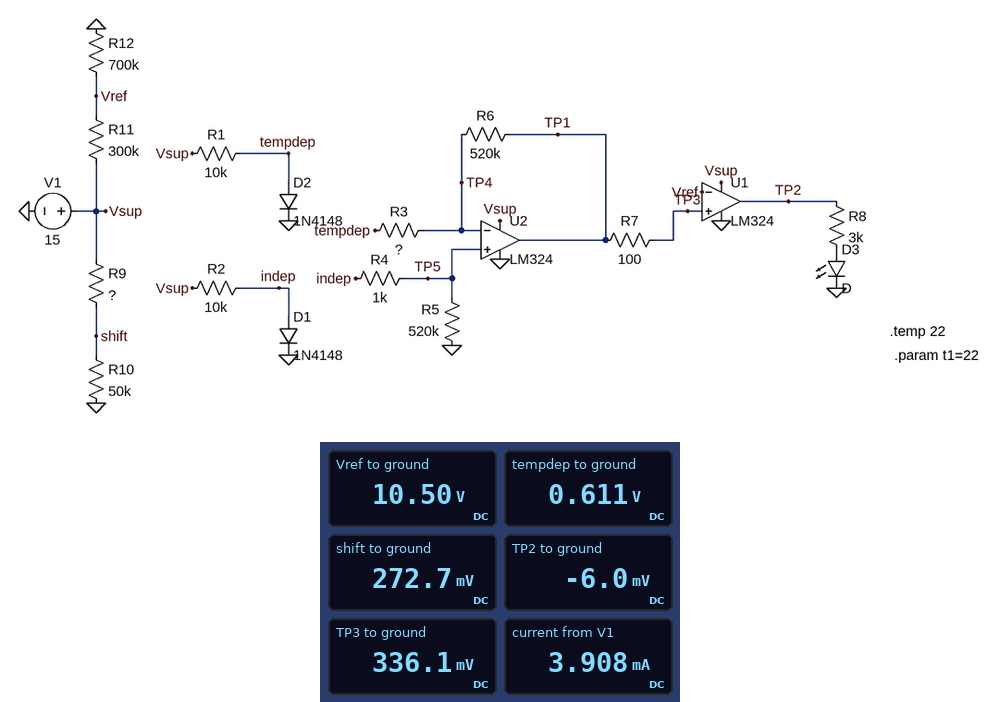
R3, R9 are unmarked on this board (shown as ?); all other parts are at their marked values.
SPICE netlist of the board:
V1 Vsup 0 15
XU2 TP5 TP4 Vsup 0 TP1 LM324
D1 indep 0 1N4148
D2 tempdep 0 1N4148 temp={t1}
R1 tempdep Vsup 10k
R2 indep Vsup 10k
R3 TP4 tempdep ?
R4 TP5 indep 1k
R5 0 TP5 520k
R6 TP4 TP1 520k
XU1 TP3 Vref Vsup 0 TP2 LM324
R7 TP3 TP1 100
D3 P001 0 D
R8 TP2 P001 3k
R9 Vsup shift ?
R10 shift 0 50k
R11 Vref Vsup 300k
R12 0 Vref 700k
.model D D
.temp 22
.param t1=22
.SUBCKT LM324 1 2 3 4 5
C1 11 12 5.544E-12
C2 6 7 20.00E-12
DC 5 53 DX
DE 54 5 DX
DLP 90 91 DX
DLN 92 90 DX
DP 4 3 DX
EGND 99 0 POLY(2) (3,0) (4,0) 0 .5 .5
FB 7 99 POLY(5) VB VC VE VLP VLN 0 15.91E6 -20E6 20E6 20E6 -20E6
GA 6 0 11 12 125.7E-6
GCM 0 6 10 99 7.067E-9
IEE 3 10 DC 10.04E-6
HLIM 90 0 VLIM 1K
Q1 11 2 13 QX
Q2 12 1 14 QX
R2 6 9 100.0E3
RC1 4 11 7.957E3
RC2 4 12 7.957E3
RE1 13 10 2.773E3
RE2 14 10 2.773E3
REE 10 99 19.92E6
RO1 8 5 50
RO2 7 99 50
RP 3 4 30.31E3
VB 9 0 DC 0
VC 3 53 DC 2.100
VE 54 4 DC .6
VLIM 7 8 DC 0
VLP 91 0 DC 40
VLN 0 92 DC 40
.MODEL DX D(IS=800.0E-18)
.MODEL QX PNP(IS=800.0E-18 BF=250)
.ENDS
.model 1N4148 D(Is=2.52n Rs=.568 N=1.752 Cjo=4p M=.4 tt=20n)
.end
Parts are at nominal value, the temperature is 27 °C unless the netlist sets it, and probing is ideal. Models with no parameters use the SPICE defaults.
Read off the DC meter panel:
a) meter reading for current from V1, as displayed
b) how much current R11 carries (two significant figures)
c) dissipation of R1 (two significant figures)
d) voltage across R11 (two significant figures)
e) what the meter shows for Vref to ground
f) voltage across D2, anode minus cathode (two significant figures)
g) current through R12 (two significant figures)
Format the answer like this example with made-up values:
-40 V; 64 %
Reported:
3.908 mA; 15 µA; 21 mW; 4.5 V; 10.50 V; 610 mV; 15 µA
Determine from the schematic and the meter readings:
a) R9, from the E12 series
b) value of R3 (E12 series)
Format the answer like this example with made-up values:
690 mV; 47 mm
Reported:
2.7 MΩ; 1.5 kΩ
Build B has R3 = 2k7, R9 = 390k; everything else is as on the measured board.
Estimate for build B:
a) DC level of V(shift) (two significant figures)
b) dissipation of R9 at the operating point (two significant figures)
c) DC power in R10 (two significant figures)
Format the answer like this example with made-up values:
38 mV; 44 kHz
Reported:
1.7 V; 450 µW; 58 µW
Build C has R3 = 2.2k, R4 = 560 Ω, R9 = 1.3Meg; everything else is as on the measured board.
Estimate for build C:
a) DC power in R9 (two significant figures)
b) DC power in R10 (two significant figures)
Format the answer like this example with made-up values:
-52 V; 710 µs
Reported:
160 µW; 6.2 µW
